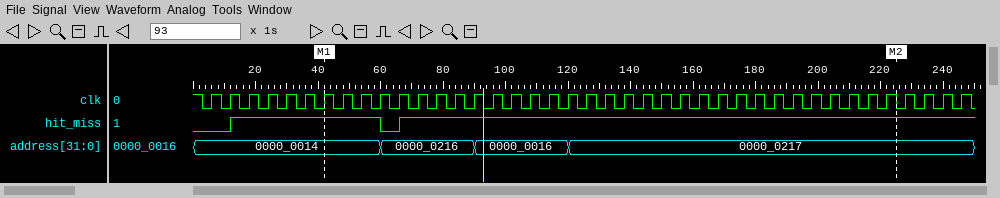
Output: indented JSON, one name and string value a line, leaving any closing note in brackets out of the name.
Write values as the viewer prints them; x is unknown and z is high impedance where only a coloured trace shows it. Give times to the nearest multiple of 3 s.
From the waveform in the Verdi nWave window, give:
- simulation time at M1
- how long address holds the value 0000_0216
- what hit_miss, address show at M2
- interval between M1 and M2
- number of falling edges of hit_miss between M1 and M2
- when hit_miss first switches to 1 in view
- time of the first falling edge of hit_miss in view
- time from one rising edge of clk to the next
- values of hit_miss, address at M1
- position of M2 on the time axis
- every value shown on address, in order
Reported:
{
  "simulation time at M1": "42 s",
  "how long address holds the value 0000_0216": "30 s",
  "what hit_miss, address show at M2": "hit_miss=1, address=0000_0217",
  "interval between M1 and M2": "183 s",
  "number of falling edges of hit_miss between M1 and M2": "1",
  "when hit_miss first switches to 1 in view": "12 s",
  "time of the first falling edge of hit_miss in view": "60 s",
  "time from one rising edge of clk to the next": "6 s",
  "values of hit_miss, address at M1": "hit_miss=1, address=0000_0014",
  "position of M2 on the time axis": "225 s",
  "every value shown on address, in order": "0000_0014, 0000_0216, 0000_0016, 0000_0217"
}
